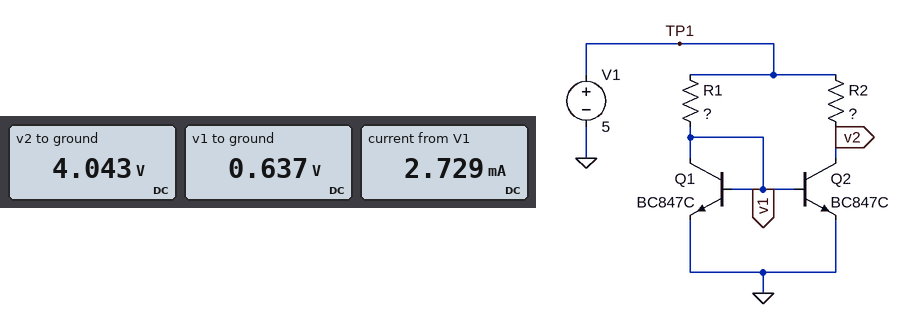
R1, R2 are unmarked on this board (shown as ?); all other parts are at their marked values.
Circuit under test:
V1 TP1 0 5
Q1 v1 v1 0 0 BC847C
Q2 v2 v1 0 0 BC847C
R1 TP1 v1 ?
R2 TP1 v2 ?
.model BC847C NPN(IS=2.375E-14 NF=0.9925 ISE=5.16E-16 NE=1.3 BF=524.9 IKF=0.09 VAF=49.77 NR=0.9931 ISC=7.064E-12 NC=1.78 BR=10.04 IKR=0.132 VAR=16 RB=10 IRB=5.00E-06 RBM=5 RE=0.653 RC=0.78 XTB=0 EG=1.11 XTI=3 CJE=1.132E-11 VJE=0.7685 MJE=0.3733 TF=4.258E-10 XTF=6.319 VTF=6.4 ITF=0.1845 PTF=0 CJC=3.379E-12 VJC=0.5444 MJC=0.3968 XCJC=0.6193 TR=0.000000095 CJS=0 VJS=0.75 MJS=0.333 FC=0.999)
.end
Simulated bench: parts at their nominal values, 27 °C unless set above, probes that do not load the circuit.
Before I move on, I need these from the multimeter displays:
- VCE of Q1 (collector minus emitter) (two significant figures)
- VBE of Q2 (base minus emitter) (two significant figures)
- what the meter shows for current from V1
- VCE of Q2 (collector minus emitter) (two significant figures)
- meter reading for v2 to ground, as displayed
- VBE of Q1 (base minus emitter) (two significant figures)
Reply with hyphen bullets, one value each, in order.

- 640 mV
- 640 mV
- 2.729 mA
- 4.0 V
- 4.043 V
- 640 mV
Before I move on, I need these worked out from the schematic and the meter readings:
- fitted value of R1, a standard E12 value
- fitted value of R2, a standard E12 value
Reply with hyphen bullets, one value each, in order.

- 3.3 kΩ
- 680 Ω
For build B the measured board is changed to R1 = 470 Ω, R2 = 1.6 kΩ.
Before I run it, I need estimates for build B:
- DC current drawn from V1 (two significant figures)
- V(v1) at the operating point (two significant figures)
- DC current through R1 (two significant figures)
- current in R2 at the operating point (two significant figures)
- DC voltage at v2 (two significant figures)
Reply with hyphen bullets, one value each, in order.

- 12 mA
- 690 mV
- 9.2 mA
- 3.1 mA
- 20 mV
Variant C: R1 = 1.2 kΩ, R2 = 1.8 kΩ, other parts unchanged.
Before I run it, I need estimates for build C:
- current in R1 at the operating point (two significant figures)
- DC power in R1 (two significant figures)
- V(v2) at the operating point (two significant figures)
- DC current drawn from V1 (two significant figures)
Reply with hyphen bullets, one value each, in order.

- 3.6 mA
- 16 mW
- 47 mV
- 6.4 mA
